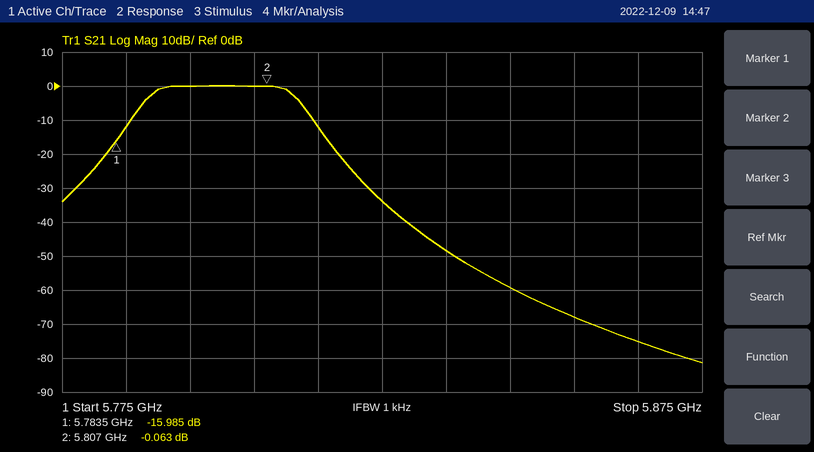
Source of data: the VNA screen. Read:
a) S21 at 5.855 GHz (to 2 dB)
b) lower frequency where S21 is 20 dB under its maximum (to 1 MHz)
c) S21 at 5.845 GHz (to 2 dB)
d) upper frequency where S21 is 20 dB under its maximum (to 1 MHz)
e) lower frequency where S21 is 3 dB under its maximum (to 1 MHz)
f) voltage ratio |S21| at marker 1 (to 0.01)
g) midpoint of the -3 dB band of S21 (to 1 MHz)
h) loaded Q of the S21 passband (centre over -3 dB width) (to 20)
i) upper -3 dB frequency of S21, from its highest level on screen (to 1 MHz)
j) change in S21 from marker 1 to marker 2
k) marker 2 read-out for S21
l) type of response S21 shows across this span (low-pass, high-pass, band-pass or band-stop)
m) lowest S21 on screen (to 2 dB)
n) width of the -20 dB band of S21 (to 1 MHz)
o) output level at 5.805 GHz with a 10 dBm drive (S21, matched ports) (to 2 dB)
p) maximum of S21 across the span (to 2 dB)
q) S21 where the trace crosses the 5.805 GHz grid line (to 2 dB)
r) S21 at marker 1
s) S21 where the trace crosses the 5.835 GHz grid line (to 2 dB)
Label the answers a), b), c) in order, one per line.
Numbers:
a) -68 dB
b) 5.782 GHz
c) -60 dB
d) 5.818 GHz
e) 5.789 GHz
f) 0.16
g) 5.800 GHz
h) 260
i) 5.811 GHz
j) 15.922 dB
k) -0.063 dB
l) band-pass
m) -82 dB
n) 36 MHz
o) 10 dBm
p) 0 dB
q) 0 dB
r) -15.985 dB
s) -48 dB
